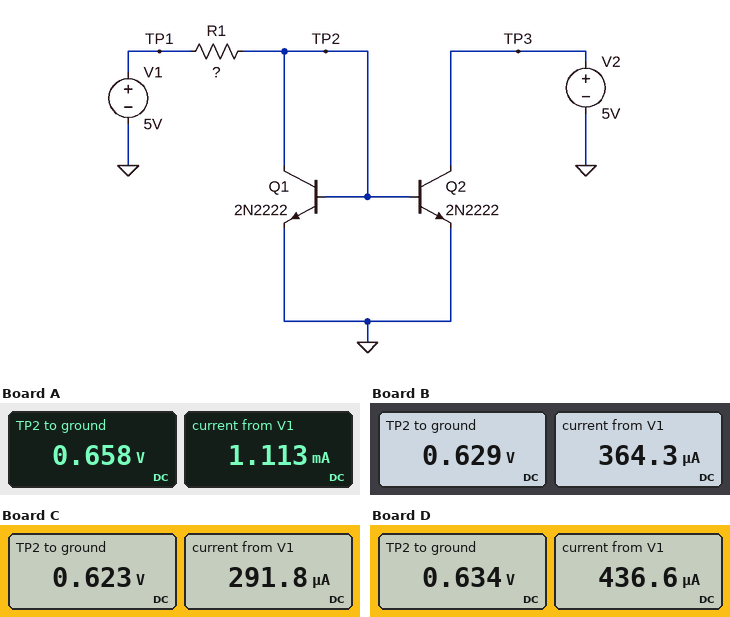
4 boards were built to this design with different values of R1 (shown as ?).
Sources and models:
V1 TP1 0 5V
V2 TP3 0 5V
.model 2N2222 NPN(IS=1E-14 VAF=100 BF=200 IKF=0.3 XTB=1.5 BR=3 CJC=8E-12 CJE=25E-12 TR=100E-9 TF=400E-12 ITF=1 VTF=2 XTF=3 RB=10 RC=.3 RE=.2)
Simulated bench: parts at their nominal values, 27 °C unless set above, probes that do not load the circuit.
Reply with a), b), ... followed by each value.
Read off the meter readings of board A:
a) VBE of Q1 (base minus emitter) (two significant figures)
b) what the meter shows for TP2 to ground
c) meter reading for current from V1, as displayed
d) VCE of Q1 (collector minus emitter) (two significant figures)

a) 660 mV
b) 0.658 V
c) 1.113 mA
d) 660 mV
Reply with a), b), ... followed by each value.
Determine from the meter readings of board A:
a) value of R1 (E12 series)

a) 3.9 kΩ
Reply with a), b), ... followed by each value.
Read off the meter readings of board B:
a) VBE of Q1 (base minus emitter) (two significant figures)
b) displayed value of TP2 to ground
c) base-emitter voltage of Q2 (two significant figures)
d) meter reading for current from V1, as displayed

a) 630 mV
b) 0.629 V
c) 630 mV
d) 364.3 µA
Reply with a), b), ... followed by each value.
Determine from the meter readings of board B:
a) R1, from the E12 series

a) 12 kΩ
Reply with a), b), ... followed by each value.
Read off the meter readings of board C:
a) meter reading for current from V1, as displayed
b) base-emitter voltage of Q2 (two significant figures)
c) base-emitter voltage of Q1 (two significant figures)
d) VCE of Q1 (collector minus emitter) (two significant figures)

a) 291.8 µA
b) 620 mV
c) 620 mV
d) 620 mV
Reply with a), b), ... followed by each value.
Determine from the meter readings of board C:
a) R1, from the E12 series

a) 15 kΩ
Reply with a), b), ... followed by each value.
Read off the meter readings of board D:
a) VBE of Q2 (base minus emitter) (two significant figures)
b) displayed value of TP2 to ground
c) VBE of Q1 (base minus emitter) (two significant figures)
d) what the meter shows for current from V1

a) 630 mV
b) 0.634 V
c) 630 mV
d) 436.6 µA
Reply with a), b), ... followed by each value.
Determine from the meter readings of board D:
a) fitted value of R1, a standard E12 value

a) 10 kΩ
